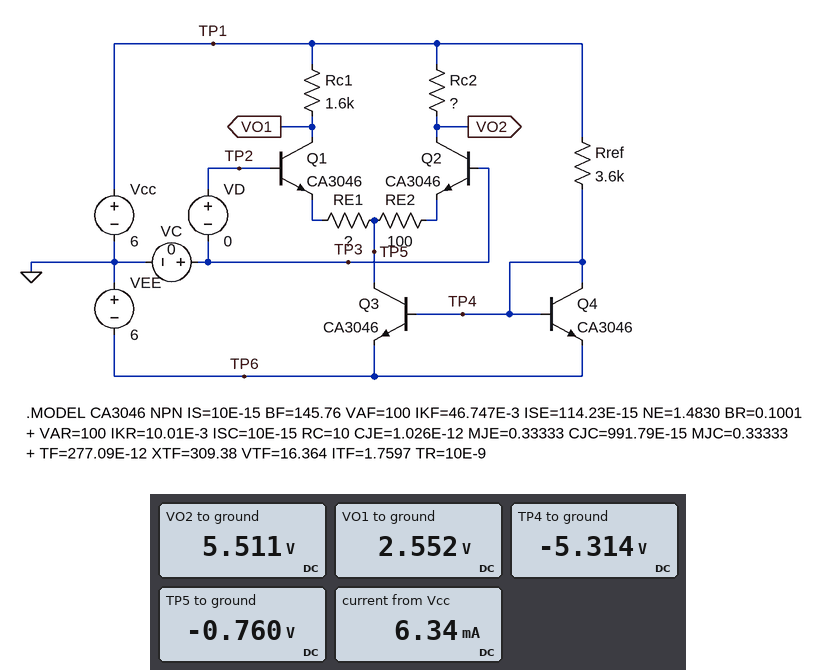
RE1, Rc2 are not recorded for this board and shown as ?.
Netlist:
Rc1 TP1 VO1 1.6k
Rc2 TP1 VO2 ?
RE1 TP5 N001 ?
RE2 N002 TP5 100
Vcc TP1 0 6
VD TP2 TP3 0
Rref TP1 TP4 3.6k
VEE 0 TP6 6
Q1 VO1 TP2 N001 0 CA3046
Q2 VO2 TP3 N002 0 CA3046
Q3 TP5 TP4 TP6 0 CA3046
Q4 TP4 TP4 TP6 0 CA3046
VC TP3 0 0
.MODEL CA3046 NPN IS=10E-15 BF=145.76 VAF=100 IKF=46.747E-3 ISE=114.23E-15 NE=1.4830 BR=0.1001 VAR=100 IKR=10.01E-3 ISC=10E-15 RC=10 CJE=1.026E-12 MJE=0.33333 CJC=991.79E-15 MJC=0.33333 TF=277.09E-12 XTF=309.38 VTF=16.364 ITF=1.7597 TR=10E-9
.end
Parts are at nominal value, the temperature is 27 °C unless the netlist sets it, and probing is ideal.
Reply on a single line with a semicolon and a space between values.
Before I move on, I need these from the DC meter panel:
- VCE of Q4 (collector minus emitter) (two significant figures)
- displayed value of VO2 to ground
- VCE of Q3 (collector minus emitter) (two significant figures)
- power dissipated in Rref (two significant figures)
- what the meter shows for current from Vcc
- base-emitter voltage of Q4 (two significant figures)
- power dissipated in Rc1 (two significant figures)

690 mV; 5.511 V; 5.2 V; 36 mW; 6.34 mA; 690 mV; 7.4 mW
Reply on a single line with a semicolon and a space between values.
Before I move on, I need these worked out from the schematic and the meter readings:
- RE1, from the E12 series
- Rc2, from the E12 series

39 Ω; 470 Ω
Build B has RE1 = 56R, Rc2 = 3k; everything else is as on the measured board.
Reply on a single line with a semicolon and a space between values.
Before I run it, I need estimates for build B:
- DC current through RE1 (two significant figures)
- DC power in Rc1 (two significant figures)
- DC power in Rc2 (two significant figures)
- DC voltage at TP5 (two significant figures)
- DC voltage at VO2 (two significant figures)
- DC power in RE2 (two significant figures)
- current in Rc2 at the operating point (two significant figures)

2.0 mA; 6.2 mW; 4.5 mW; -780 mV; 2.3 V; 150 µW; 1.2 mA
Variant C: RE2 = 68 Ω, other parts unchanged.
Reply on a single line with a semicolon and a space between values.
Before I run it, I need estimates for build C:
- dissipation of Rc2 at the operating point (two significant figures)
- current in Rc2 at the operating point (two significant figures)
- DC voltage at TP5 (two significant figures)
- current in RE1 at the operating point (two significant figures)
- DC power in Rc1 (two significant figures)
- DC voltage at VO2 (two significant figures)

760 µW; 1.3 mA; -750 mV; 1.9 mA; 5.9 mW; 5.4 V
